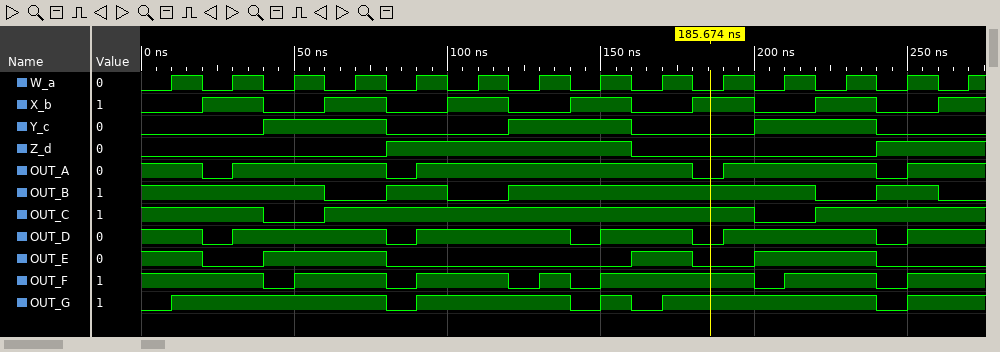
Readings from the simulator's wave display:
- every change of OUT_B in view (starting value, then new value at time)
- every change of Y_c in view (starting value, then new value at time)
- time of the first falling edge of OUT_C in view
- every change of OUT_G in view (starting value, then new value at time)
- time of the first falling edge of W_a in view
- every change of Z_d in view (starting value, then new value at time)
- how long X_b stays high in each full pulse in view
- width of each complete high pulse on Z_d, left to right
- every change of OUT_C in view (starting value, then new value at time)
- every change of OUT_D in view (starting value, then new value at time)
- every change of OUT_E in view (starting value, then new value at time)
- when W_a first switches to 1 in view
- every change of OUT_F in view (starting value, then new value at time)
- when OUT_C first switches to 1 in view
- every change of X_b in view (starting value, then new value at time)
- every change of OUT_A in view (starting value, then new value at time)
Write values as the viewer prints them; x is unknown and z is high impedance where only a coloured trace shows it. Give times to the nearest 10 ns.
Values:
1, 0 at 60 ns, 1 at 80 ns, 0 at 100 ns, 1 at 120 ns, 0 at 220 ns, 1 at 240 ns, 0 at 260 ns
0, 1 at 40 ns, 0 at 80 ns, 1 at 120 ns, 0 at 160 ns, 1 at 200 ns, 0 at 240 ns
40 ns
0, 1 at 10 ns, 0 at 80 ns, 1 at 90 ns, 0 at 140 ns, 1 at 150 ns, 0 at 160 ns, 1 at 170 ns, 0 at 240 ns, 1 at 250 ns
20 ns
0, 1 at 80 ns, 0 at 160 ns, 1 at 240 ns
20 ns, 20 ns, 20 ns, 20 ns, 20 ns, 20 ns
80 ns
1, 0 at 40 ns, 1 at 60 ns, 0 at 200 ns, 1 at 220 ns
1, 0 at 20 ns, 1 at 30 ns, 0 at 80 ns, 1 at 90 ns, 0 at 140 ns, 1 at 150 ns, 0 at 180 ns, 1 at 190 ns, 0 at 240 ns, 1 at 250 ns
1, 0 at 20 ns, 1 at 40 ns, 0 at 80 ns, 1 at 160 ns, 0 at 180 ns, 1 at 200 ns, 0 at 240 ns
10 ns
1, 0 at 40 ns, 1 at 50 ns, 0 at 80 ns, 1 at 90 ns, 0 at 120 ns, 1 at 130 ns, 0 at 140 ns, 1 at 150 ns, 0 at 200 ns, 1 at 210 ns, 0 at 240 ns, 1 at 250 ns
60 ns
0, 1 at 20 ns, 0 at 40 ns, 1 at 60 ns, 0 at 80 ns, 1 at 100 ns, 0 at 120 ns, 1 at 140 ns, 0 at 160 ns, 1 at 180 ns, 0 at 200 ns, 1 at 220 ns, 0 at 240 ns, 1 at 260 ns
1, 0 at 20 ns, 1 at 30 ns, 0 at 80 ns, 1 at 90 ns, 0 at 180 ns, 1 at 190 ns, 0 at 240 ns, 1 at 250 ns
